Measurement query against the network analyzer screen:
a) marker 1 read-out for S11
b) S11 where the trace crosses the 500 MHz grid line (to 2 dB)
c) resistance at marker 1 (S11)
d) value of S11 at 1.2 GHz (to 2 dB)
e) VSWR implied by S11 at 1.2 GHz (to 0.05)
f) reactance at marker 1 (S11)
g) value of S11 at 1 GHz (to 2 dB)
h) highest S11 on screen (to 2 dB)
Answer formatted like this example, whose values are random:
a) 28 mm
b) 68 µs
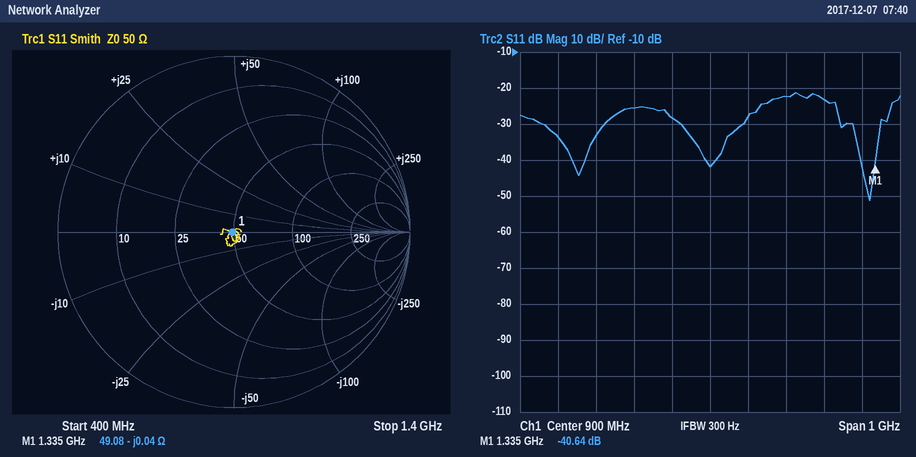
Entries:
a) -40.64 dB
b) -34 dB
c) 49.08 Ω
d) -24 dB
e) 1.15
f) -0.04 Ω
g) -28 dB
h) -22 dB
